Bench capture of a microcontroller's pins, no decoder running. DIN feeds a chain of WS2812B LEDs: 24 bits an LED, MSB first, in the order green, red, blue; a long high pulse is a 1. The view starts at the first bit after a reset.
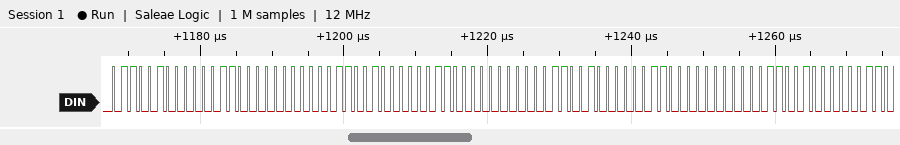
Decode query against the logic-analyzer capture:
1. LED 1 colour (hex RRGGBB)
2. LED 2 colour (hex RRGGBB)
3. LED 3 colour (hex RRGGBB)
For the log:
#0C6400
#0C6400
#0C6400
